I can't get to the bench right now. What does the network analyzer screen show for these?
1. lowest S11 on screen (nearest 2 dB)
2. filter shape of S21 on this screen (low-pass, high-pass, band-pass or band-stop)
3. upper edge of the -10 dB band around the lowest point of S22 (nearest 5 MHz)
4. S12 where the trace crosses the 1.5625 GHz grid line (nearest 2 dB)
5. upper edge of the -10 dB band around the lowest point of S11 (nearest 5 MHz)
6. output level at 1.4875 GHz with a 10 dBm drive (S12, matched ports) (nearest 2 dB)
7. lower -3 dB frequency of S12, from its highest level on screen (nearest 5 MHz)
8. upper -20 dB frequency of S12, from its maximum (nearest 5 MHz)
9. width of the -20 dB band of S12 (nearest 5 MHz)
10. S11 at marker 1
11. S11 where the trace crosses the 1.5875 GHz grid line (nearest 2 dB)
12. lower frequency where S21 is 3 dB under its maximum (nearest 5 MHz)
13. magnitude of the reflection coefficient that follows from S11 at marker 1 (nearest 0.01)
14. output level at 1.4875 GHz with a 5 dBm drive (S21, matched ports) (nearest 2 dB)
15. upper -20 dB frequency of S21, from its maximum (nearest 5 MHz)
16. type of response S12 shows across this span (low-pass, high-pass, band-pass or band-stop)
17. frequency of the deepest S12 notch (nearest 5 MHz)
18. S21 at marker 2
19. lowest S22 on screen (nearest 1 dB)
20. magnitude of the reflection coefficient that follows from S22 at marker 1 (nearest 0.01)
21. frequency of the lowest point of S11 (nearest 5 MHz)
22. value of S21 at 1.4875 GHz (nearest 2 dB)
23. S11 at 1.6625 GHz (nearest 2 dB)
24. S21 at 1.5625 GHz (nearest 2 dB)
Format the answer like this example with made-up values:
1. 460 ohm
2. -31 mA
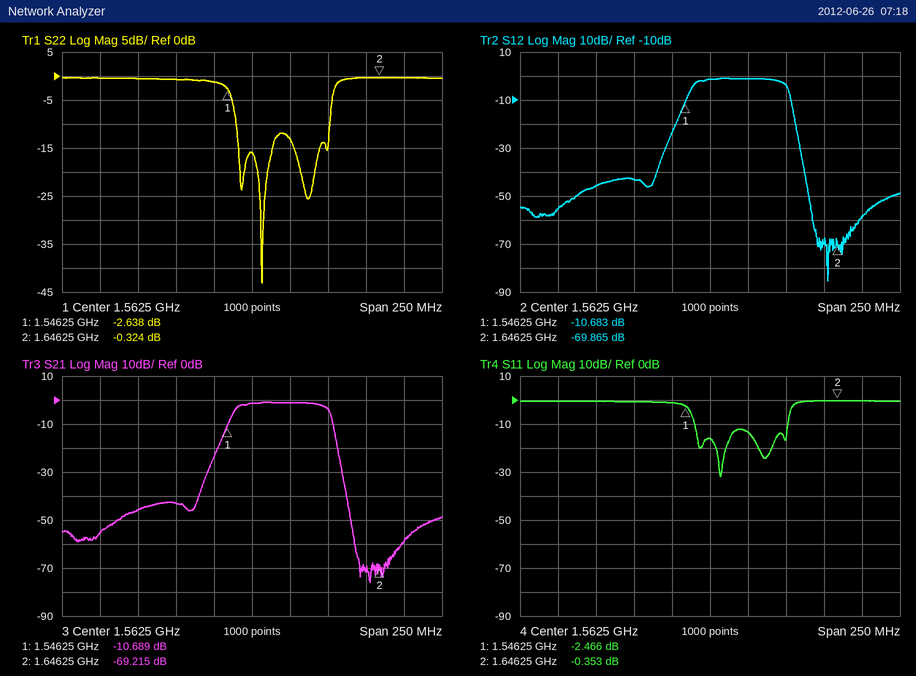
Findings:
1. -32 dB
2. band-pass
3. 1.615 GHz
4. -2 dB
5. 1.615 GHz
6. -36 dBm
7. 1.550 GHz
8. 1.620 GHz
9. 80 MHz
10. -2.466 dB
11. -14 dB
12. 1.550 GHz
13. 0.75
14. -40 dBm
15. 1.620 GHz
16. band-pass
17. 1.640 GHz
18. -69.215 dB
19. -43 dB
20. 0.74
21. 1.570 GHz
22. -46 dB
23. 0 dB
24. -2 dB
